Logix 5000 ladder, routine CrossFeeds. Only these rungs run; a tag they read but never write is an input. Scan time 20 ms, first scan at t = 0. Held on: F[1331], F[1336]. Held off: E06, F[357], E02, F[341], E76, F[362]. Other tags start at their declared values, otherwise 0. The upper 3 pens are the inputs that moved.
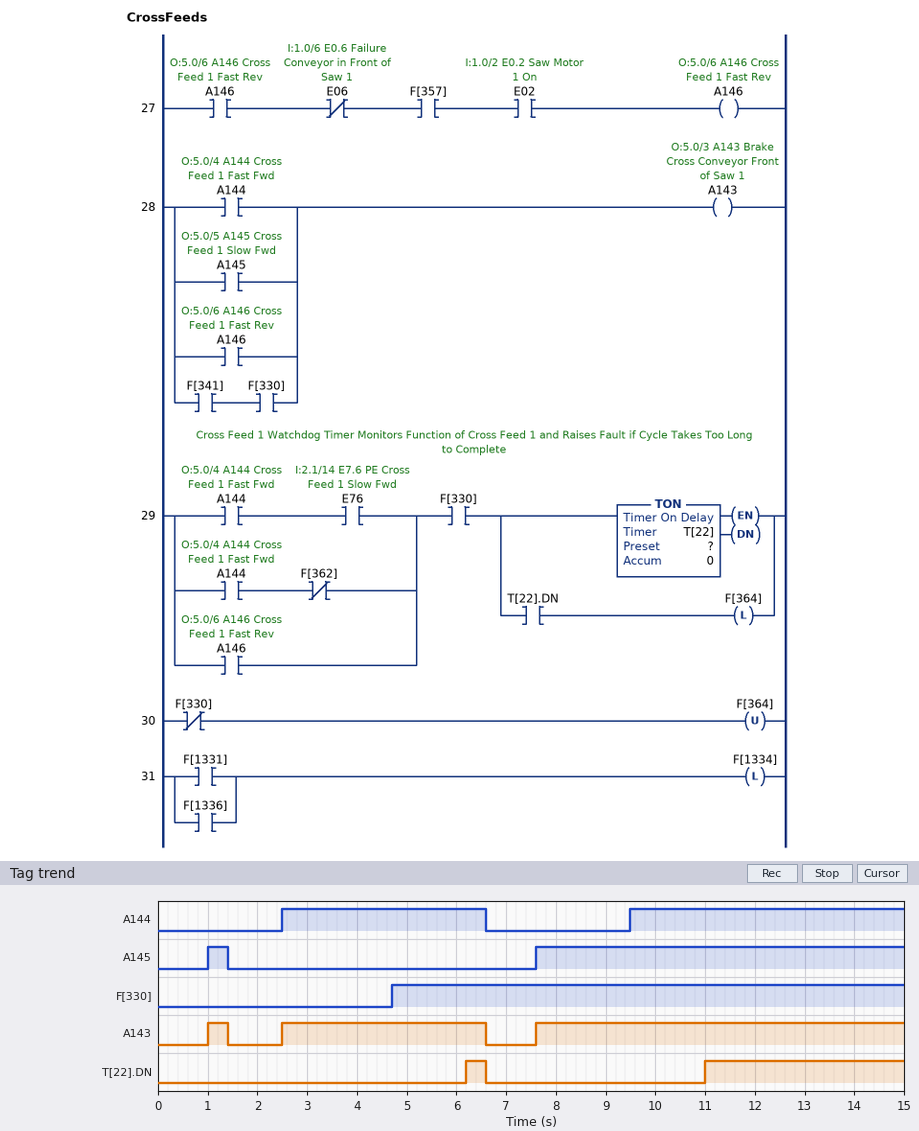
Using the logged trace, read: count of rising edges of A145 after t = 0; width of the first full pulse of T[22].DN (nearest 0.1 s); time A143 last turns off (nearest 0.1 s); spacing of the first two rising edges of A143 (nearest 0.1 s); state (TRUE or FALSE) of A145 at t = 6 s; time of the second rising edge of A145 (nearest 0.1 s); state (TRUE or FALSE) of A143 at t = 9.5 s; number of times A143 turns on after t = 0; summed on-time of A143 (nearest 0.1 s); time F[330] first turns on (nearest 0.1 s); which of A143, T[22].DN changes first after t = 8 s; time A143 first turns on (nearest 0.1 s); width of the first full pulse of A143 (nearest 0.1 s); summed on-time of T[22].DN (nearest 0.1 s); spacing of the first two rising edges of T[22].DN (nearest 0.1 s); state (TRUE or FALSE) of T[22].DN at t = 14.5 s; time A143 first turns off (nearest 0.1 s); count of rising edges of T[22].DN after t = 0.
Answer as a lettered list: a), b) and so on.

a) 2
b) 0.4 s
c) 6.6 s
d) 1.5 s
e) FALSE
f) 7.6 s
g) TRUE
h) 3
i) 11.9 s
j) 4.7 s
k) T[22].DN
l) 1.0 s
m) 0.4 s
n) 4.4 s
o) 4.8 s
p) TRUE
q) 1.4 s
r) 2
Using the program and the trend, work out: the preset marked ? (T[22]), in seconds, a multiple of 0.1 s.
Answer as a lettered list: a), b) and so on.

a) 1.5 s
